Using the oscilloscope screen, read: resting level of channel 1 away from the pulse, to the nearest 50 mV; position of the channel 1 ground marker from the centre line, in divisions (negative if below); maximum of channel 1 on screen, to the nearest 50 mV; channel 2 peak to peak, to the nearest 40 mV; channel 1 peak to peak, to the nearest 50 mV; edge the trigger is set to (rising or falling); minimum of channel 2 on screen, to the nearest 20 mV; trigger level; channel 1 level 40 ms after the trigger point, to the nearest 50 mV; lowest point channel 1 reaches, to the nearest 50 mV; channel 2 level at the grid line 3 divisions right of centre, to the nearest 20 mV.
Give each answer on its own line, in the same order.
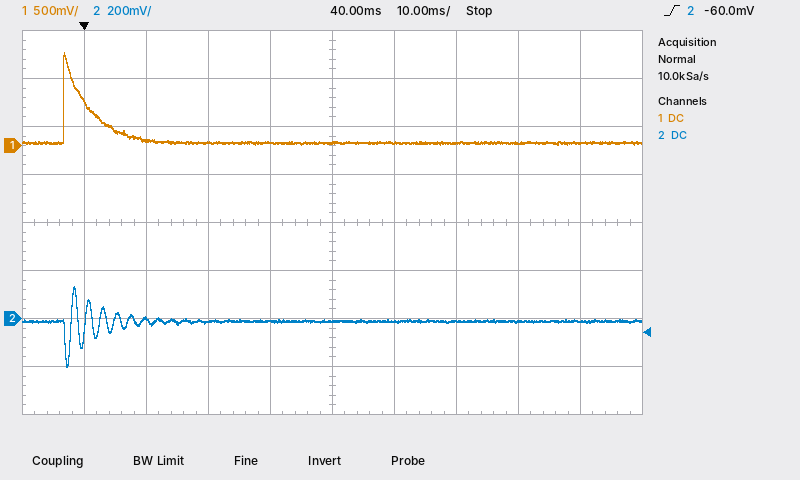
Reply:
50 mV
+1.6 div
950 mV
320 mV
950 mV
rising
-200 mV
-60.0 mV
50 mV
0 mV
-20 mV
